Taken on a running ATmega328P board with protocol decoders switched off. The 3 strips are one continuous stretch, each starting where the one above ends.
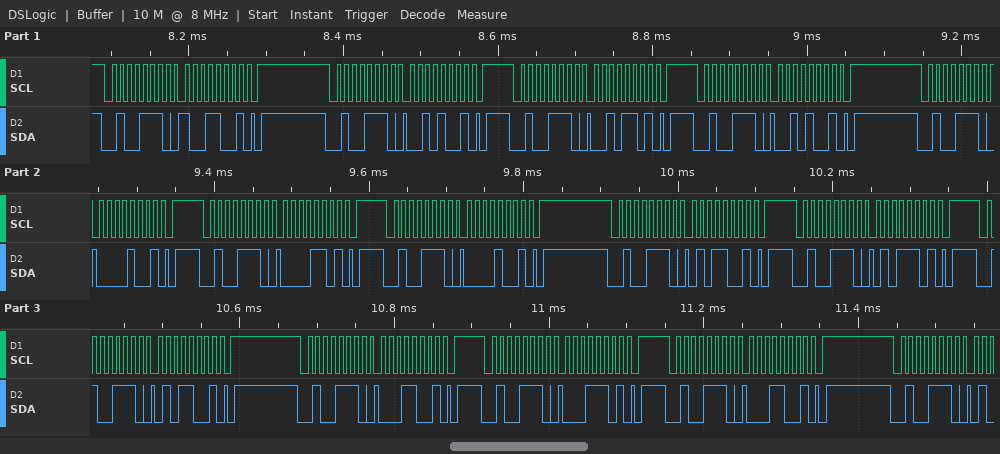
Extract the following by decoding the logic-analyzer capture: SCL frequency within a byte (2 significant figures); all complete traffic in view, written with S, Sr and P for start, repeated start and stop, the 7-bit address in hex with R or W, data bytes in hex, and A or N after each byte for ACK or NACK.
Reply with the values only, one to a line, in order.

100 kHz
S 27W A 99 A P S 27W A 29 A P S 27W A 2D A P S 27W A 29 A P S 27W A 09 A P S 27W A 0D A P S 27W A 09 A P S 27W A 59 A P S 27W A 5D A P S 27W A 59 A P S 27W A 19 A P S 27W A 1D A P S 27W A 19 A P S 27W A
